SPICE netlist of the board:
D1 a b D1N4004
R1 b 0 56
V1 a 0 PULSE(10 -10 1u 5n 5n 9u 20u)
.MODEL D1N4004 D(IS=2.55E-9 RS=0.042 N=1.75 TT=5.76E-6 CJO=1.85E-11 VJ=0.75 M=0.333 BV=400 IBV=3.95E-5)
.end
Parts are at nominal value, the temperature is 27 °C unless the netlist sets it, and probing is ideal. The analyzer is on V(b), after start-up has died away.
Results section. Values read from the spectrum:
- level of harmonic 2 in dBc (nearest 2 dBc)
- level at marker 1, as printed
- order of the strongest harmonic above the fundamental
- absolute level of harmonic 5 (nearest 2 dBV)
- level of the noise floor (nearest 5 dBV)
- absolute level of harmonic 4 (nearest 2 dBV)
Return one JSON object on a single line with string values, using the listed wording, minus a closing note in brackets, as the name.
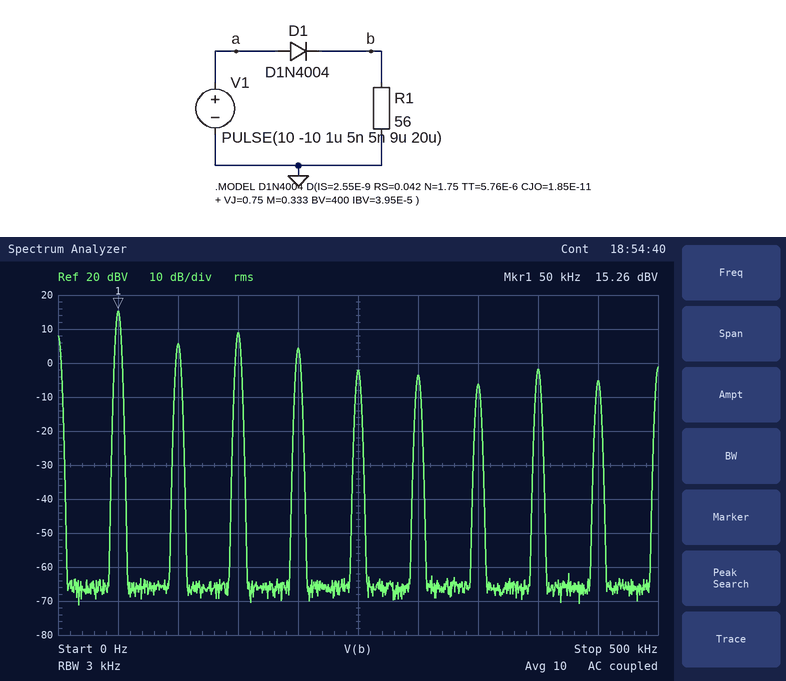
{"level of harmonic 2 in dBc": "-10 dBc", "level at marker 1, as printed": "15.26 dBV", "order of the strongest harmonic above the fundamental": "3", "absolute level of harmonic 5": "-2 dBV", "level of the noise floor": "-65 dBV", "absolute level of harmonic 4": "4 dBV"}
